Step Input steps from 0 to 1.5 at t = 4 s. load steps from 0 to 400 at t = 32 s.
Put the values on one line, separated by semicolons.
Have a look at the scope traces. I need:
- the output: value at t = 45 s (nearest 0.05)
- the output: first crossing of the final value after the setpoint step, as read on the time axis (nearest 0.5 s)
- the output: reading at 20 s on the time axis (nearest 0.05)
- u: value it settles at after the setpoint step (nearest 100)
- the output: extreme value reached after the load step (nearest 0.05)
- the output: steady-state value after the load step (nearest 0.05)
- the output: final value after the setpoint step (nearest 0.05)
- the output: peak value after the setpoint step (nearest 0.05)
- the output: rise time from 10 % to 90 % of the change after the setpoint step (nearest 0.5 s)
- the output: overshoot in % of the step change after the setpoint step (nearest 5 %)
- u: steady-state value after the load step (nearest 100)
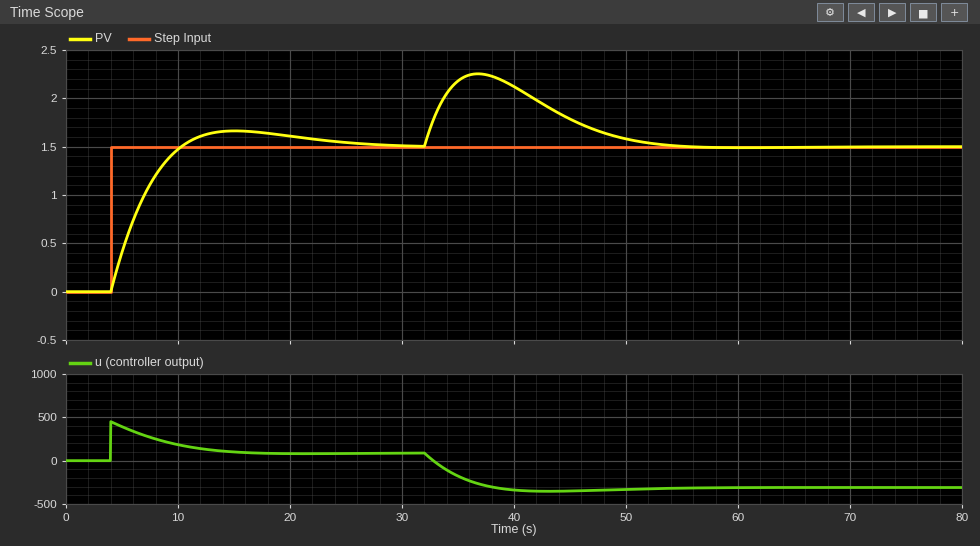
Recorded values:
1.80; 10.5 s; 1.60; 100; 2.25; 1.50; 1.50; 1.65; 4.5 s; 10 %; -300
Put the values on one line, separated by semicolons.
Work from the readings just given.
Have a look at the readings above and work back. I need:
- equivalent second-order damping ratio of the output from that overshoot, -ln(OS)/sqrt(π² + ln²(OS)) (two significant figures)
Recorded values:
0.59
